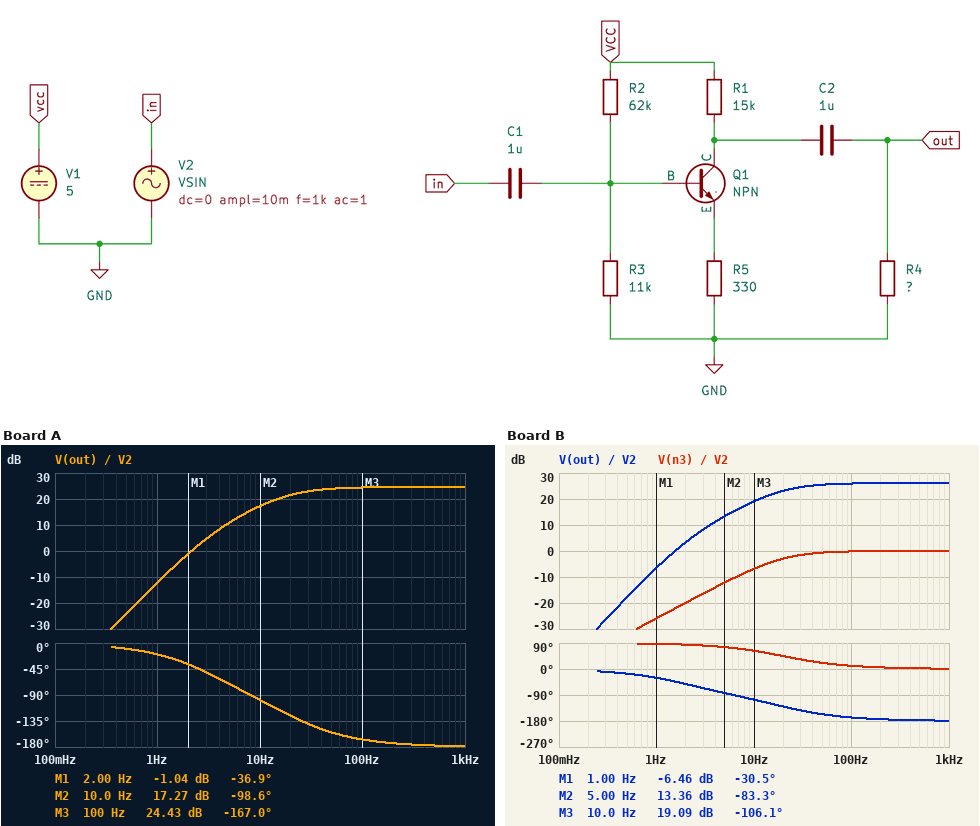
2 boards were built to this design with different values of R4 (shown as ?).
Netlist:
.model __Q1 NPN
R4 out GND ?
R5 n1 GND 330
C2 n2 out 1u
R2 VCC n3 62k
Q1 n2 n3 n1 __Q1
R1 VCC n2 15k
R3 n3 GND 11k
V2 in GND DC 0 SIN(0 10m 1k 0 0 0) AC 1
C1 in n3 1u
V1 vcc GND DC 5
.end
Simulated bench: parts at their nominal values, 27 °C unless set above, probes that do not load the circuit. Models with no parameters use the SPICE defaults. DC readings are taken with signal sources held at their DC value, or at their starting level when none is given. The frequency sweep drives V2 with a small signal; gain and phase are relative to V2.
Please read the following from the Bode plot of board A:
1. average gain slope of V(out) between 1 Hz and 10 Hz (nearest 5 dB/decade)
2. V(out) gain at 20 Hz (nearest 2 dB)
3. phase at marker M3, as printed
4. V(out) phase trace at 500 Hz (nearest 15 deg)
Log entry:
30 dB/decade
22 dB
-167.0 deg
-180 deg
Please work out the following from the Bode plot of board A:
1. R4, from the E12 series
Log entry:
33 kΩ
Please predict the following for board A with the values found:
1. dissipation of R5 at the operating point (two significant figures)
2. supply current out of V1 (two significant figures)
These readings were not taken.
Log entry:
3.0 µW
160 µA
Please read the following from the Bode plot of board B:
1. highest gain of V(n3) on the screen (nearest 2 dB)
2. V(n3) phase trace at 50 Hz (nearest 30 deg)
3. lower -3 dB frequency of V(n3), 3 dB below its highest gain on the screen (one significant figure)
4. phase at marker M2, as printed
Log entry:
0 dB
30 deg
20 Hz
-83.3 deg
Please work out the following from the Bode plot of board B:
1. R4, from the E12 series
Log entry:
68 kΩ
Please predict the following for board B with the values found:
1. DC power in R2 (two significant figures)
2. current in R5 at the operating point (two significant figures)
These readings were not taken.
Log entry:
290 µW
95 µA
